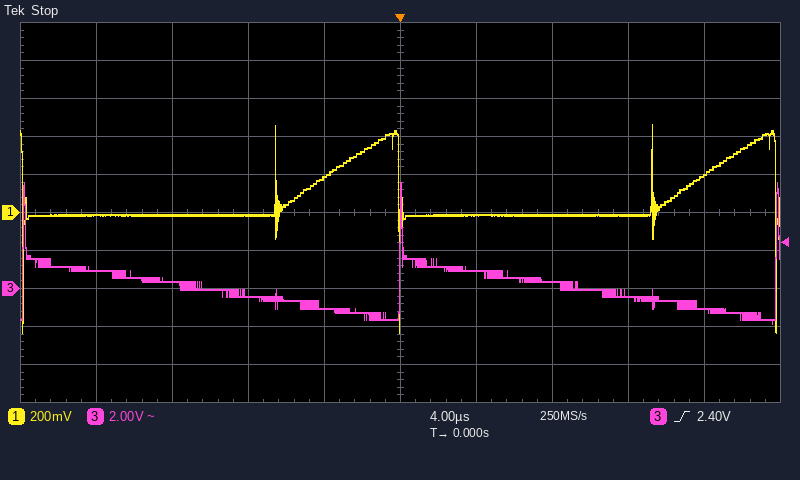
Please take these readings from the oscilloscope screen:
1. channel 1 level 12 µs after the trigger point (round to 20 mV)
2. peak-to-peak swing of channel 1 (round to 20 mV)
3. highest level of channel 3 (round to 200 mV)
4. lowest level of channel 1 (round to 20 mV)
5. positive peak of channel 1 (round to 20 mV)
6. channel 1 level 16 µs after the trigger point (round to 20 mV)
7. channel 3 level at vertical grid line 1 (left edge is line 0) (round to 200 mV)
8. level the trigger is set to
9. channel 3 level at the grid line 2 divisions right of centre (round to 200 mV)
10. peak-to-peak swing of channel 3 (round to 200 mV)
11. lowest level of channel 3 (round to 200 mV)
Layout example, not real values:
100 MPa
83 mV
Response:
-20 mV
1.10 V
5.6 V
-640 mV
460 mV
200 mV
1.0 V
2.40 V
400 mV
7.4 V
-1.8 V
